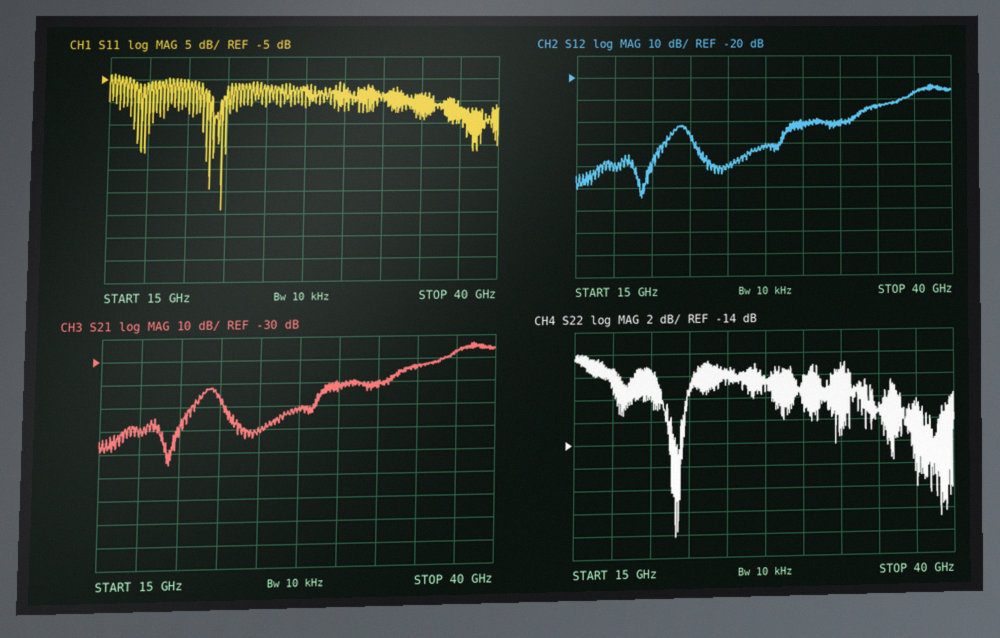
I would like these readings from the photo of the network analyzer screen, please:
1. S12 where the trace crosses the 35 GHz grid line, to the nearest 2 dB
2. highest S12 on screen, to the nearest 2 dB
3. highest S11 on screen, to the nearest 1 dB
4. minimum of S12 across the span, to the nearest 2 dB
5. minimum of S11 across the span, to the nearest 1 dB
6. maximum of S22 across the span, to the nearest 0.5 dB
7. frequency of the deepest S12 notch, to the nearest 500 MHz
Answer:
-34 dB
-24 dB
-4 dB
-74 dB
-34 dB
-6.0 dB
19.5 GHz
